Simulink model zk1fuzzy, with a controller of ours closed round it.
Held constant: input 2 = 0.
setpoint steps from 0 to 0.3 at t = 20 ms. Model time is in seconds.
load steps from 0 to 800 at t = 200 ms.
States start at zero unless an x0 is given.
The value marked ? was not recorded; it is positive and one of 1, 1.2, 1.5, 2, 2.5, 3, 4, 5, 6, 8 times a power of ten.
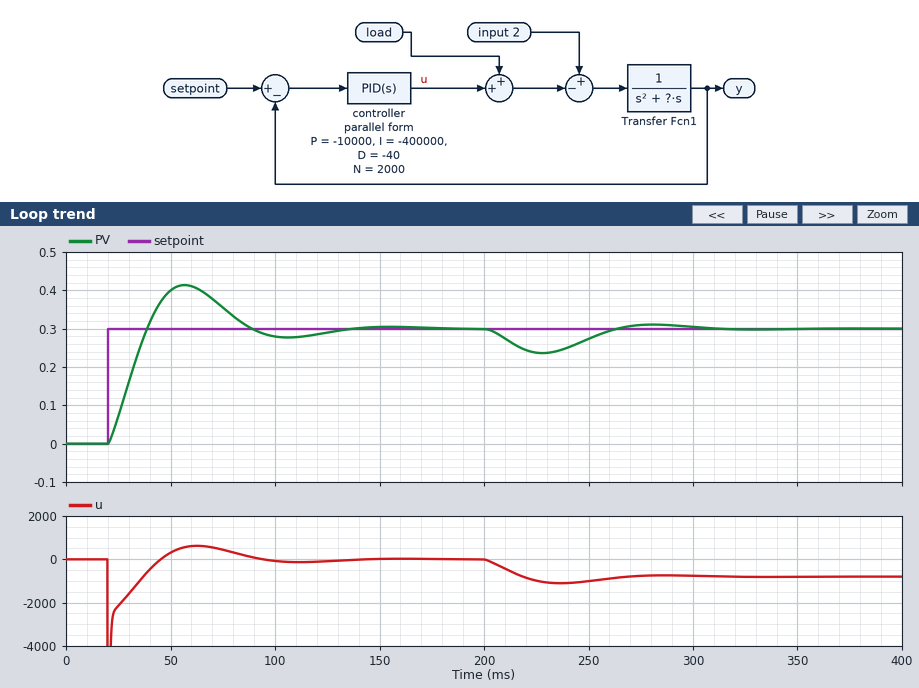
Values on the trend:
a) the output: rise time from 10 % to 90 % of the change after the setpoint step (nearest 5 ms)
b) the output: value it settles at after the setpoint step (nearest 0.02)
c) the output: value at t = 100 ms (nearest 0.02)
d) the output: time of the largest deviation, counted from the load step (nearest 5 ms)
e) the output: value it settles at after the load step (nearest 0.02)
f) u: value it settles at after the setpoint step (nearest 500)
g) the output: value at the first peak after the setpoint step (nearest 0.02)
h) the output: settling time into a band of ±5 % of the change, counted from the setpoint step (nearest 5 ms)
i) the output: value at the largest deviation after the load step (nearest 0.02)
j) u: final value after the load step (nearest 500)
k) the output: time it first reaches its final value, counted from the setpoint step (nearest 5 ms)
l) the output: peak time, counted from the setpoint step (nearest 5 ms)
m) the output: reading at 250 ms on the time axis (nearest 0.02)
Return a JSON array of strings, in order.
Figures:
["15 ms", "0.30", "0.28", "30 ms", "0.30", "0", "0.42", "100 ms", "0.24", "-1000", "20 ms", "35 ms", "0.28"]
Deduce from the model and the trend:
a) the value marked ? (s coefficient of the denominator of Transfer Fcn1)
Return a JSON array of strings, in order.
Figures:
["100"]
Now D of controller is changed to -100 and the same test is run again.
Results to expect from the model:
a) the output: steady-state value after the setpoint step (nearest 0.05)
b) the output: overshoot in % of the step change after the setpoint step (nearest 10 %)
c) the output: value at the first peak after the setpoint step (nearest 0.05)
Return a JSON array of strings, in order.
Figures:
["0.30", "20 %", "0.35"]
